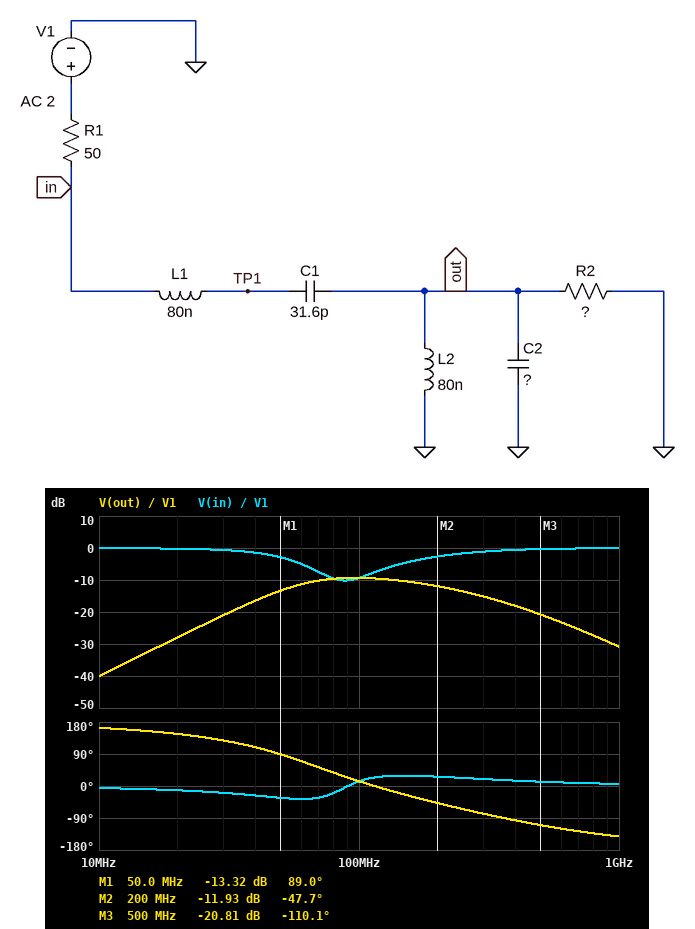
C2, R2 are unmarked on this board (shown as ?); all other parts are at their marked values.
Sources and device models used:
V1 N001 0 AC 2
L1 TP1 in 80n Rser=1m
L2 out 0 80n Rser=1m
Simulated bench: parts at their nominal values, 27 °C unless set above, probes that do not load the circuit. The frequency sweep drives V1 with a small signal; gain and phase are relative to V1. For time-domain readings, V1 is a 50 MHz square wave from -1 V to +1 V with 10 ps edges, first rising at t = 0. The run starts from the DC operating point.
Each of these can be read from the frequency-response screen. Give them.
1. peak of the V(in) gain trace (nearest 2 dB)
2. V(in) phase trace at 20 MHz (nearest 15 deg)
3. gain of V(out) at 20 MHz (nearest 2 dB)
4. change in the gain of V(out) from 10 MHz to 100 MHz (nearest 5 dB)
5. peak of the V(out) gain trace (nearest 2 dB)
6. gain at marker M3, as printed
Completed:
0 dB
-15 deg
-28 dB
30 dB
-10 dB
-20.81 dB
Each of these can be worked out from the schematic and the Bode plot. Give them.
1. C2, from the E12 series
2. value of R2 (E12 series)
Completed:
10 pF
27 Ω
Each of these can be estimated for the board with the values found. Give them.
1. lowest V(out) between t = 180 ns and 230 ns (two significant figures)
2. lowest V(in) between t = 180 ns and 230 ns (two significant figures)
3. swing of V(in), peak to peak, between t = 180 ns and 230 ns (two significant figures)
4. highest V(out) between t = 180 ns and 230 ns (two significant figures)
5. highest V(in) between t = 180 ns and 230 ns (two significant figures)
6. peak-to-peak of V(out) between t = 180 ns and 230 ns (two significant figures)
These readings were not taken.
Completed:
-430 mV
-1.1 V
2.2 V
430 mV
1.1 V
870 mV
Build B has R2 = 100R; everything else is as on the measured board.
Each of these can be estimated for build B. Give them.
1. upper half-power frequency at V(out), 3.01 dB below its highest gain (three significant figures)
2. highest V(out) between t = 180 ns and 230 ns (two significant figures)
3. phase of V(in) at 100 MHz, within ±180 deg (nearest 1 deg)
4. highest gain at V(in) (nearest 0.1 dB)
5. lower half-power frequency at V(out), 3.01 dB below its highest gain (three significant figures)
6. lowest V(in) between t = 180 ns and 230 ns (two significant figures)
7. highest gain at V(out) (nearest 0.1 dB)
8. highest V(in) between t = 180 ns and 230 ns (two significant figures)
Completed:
319 MHz
750 mV
24 deg
0 dB
57.0 MHz
-1.2 V
-3.8 dB
1.2 V
